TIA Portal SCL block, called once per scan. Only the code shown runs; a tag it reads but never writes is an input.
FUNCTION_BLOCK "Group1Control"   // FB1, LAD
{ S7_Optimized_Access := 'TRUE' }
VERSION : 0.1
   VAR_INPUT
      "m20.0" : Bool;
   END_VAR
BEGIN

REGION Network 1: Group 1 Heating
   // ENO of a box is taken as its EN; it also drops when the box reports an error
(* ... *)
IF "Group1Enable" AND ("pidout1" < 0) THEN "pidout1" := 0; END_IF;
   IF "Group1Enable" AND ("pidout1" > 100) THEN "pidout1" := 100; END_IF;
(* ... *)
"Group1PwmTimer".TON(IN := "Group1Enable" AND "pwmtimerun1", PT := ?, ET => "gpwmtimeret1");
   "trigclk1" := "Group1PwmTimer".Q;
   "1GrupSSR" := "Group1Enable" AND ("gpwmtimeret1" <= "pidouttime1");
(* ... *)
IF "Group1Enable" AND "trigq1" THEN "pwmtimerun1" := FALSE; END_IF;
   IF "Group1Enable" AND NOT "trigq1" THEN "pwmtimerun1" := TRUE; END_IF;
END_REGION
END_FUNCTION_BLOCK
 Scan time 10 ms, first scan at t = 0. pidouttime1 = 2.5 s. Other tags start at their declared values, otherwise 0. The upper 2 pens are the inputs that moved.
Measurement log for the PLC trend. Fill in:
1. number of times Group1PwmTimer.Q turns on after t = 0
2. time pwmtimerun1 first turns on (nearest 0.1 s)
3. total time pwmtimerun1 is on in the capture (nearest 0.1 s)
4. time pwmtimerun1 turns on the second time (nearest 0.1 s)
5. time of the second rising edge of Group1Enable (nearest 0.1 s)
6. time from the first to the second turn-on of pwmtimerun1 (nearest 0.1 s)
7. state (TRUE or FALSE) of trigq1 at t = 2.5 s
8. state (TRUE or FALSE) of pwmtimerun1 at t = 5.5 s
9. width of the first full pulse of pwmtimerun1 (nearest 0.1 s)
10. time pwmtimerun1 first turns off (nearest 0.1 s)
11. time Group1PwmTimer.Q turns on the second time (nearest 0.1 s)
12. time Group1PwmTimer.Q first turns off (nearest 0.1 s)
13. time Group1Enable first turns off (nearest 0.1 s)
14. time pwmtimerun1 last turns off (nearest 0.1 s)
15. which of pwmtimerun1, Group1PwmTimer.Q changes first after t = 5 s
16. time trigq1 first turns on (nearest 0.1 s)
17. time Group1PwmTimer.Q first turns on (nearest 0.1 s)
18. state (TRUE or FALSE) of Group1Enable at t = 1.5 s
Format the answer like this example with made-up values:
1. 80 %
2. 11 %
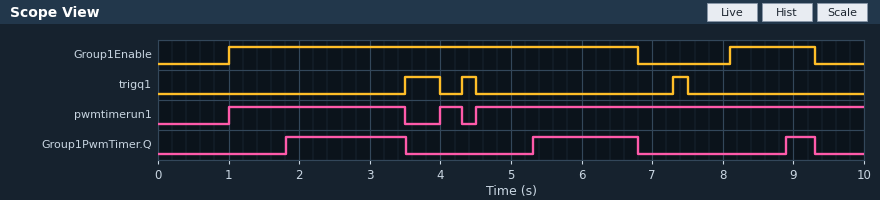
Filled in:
1. 3
2. 1.0 s
3. 8.3 s
4. 4.0 s
5. 8.1 s
6. 3.0 s
7. FALSE
8. TRUE
9. 2.5 s
10. 3.5 s
11. 5.3 s
12. 3.5 s
13. 6.8 s
14. 4.3 s
15. Group1PwmTimer.Q
16. 3.5 s
17. 1.8 s
18. TRUE
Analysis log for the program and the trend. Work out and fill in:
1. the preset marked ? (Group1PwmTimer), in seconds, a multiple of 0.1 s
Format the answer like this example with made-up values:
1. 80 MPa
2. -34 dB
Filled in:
1. 0.8 s
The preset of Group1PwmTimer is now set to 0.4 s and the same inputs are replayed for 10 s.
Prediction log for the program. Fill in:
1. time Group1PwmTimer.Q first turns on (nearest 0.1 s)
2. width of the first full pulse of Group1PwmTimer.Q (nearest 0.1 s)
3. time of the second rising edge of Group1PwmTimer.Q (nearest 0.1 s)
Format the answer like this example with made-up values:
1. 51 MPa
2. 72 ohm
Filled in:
1. 1.4 s
2. 2.1 s
3. 4.9 s
